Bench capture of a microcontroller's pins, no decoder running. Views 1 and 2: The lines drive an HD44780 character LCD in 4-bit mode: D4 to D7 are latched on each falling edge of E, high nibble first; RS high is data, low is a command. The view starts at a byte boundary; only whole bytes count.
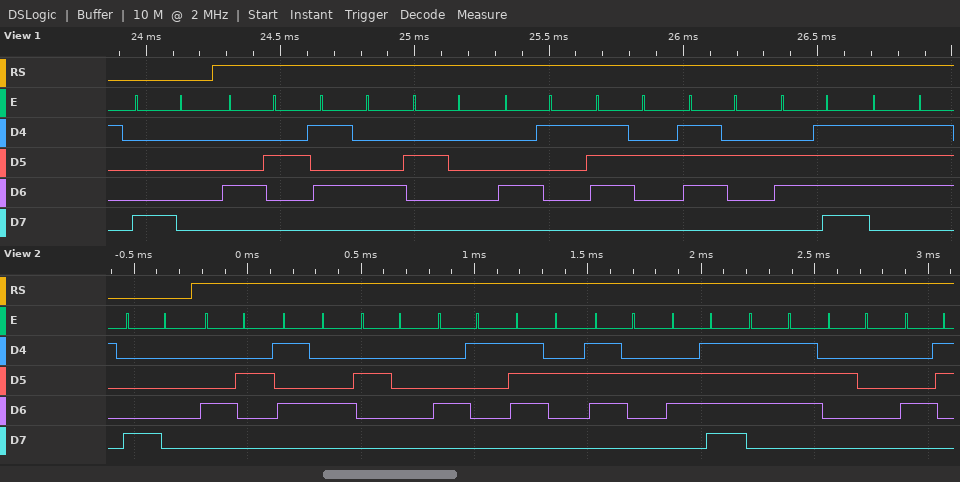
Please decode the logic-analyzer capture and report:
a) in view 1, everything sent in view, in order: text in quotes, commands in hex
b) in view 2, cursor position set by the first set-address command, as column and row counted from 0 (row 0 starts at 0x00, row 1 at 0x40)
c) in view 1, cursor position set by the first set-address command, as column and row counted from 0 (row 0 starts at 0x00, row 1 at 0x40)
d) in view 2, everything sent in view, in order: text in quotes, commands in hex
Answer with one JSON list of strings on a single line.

["0x80 \"BT Arrow\"", "column 0, row 0", "column 0, row 0", "0x80 \"BT Arrow C\""]
